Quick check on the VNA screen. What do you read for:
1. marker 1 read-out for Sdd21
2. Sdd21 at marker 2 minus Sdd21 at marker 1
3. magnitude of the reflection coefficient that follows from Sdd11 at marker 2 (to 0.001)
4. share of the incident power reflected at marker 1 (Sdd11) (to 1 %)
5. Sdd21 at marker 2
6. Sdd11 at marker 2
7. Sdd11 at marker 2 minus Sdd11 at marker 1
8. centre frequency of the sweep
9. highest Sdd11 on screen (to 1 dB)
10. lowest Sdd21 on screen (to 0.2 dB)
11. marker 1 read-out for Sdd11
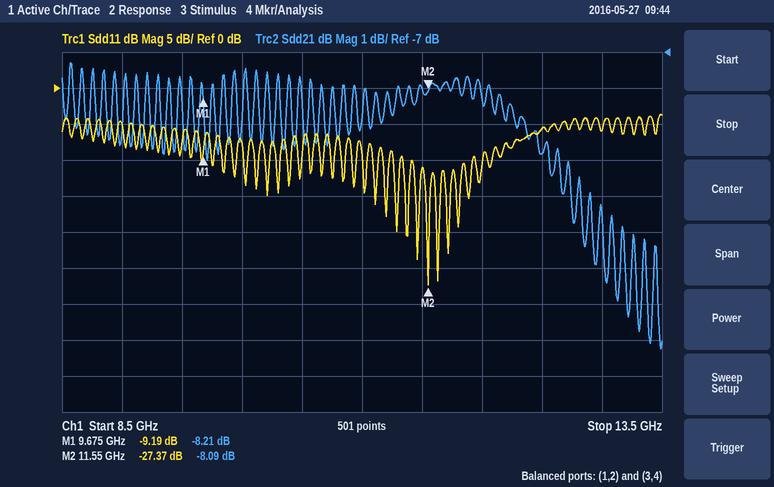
-8.21 dB
0.12 dB
0.043
12 %
-8.09 dB
-27.37 dB
-18.18 dB
11 GHz
-4 dB
-15.2 dB
-9.19 dB
